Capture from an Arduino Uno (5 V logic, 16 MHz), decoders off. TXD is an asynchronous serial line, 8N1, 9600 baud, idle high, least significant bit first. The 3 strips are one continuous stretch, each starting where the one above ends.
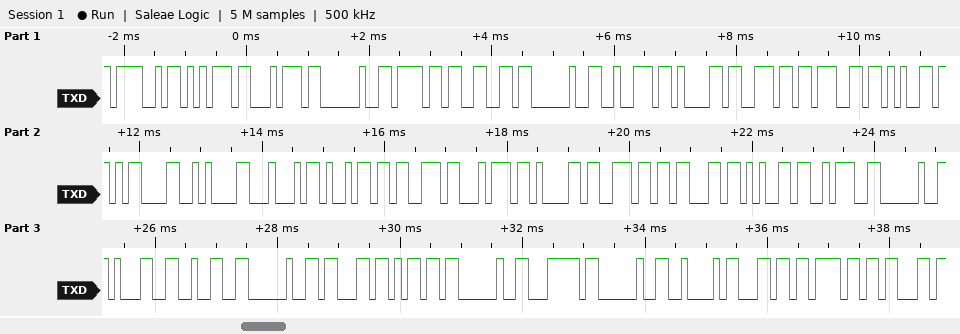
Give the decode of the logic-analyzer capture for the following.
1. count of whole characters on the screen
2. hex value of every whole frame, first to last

36
4F 75 74 20 6F 66 20 72 61 6E 67 65 0D 0A 44 69 73 74 61 6E 63 65 3A 20 31 32 20 63 6D 20 7C 20 42 6C 6F 63
